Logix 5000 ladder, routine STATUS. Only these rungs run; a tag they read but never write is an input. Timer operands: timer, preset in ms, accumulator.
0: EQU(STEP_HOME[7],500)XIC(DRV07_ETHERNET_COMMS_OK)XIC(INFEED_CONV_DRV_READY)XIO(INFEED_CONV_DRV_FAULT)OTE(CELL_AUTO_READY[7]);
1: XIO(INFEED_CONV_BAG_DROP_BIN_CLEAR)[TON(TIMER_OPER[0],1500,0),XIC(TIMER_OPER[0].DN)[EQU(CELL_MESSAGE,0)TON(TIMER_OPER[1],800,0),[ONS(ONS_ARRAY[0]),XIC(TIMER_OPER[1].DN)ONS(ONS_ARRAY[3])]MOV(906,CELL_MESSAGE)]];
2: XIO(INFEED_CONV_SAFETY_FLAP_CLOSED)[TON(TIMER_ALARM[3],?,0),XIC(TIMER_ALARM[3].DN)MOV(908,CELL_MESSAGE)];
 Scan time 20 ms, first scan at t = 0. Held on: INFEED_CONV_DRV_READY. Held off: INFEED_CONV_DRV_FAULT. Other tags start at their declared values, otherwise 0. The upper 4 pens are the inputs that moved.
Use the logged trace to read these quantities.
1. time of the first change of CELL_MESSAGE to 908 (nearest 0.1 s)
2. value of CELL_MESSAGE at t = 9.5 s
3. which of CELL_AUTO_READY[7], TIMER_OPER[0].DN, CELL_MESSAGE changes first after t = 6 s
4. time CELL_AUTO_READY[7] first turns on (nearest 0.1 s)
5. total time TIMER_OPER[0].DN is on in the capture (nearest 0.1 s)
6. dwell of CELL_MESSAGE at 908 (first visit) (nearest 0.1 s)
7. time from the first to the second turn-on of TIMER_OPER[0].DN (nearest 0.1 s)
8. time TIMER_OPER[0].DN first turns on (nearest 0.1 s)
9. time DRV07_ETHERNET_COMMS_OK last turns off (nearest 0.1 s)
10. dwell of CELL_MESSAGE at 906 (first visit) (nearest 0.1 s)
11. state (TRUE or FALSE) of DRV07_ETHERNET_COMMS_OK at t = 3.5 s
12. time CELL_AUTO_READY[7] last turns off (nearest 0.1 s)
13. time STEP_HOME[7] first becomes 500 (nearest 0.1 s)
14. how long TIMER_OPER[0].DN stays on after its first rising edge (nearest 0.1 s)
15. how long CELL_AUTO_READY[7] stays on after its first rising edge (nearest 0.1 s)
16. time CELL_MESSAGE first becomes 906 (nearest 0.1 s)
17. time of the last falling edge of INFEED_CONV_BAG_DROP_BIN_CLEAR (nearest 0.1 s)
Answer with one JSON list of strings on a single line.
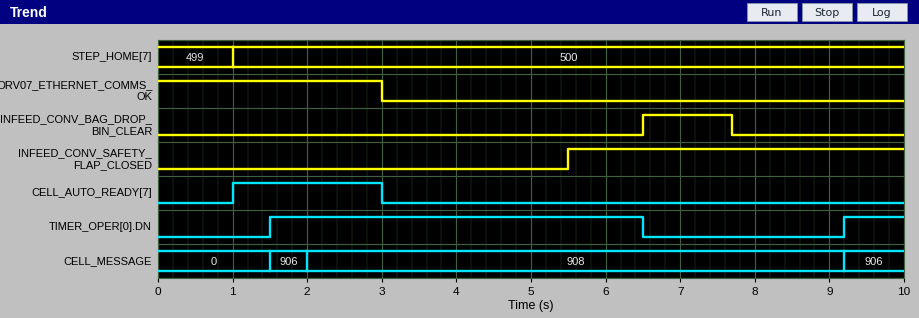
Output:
["2.0 s", "906", "TIMER_OPER[0].DN", "1.0 s", "5.8 s", "7.2 s", "7.7 s", "1.5 s", "3.0 s", "0.5 s", "FALSE", "3.0 s", "1.0 s", "5.0 s", "2.0 s", "1.5 s", "7.7 s"]
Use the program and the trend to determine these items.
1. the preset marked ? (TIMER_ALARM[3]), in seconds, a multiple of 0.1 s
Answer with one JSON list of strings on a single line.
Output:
["2.0 s"]
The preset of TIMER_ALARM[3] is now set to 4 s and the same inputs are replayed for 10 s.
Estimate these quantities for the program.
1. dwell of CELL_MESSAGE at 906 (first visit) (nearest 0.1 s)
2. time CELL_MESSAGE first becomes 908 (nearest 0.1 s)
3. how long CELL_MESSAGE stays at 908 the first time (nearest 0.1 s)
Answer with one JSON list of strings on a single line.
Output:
["2.5 s", "4.0 s", "5.2 s"]
